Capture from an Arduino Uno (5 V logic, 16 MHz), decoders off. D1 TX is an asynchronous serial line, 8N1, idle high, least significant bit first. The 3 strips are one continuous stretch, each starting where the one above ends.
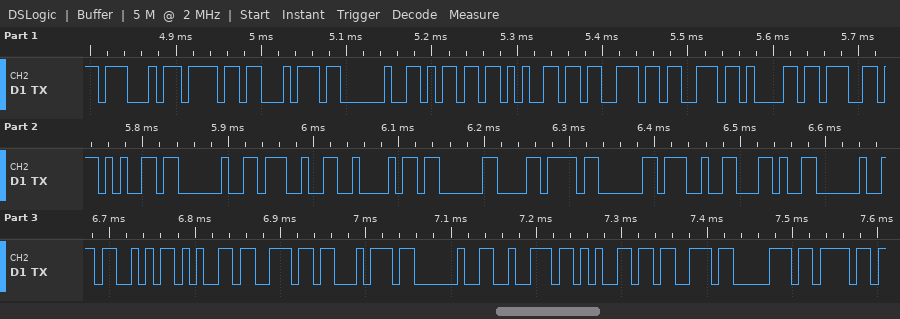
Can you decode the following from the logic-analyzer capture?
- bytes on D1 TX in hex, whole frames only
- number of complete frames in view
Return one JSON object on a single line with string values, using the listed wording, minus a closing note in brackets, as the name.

{"bytes on D1 TX in hex, whole frames only": "47 6F 74 20 6D 65 73 73 61 67 65 20 27 42 03 D8 03 27 2C 20 53 65 6E 74 20 72 65 73 70 6F", "number of complete frames in view": "30"}
